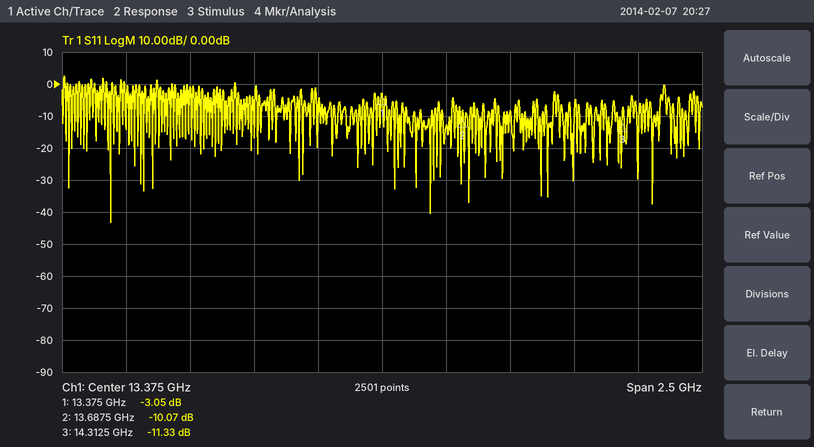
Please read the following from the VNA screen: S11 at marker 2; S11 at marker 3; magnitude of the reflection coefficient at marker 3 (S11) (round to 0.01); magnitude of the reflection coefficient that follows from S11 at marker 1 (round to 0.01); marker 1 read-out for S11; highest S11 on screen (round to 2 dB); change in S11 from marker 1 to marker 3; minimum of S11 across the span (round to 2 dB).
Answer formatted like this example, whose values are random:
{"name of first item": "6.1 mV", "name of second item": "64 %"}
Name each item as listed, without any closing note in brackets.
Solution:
{"S11 at marker 2": "-10.07 dB", "S11 at marker 3": "-11.33 dB", "magnitude of the reflection coefficient at marker 3 (S11)": "0.27", "magnitude of the reflection coefficient that follows from S11 at marker 1": "0.70", "marker 1 read-out for S11": "-3.05 dB", "highest S11 on screen": "2 dB", "change in S11 from marker 1 to marker 3": "-8.28 dB", "minimum of S11 across the span": "-44 dB"}
